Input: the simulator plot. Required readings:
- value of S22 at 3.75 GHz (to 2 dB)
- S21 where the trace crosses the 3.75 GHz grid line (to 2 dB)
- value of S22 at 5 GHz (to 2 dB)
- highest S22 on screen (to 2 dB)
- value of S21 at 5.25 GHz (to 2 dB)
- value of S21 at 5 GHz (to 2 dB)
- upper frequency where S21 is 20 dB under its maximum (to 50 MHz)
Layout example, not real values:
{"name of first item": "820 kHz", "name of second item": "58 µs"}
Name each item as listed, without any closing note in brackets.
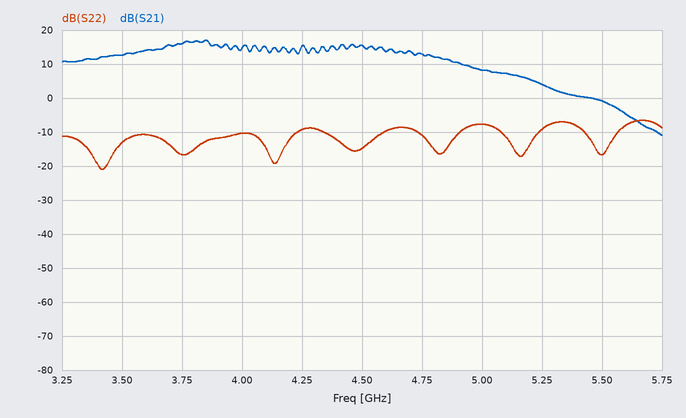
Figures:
{"value of S22 at 3.75 GHz": "-16 dB", "S21 where the trace crosses the 3.75 GHz grid line": "16 dB", "value of S22 at 5 GHz": "-8 dB", "highest S22 on screen": "-6 dB", "value of S21 at 5.25 GHz": "4 dB", "value of S21 at 5 GHz": "8 dB", "upper frequency where S21 is 20 dB under its maximum": "5.55 GHz"}
